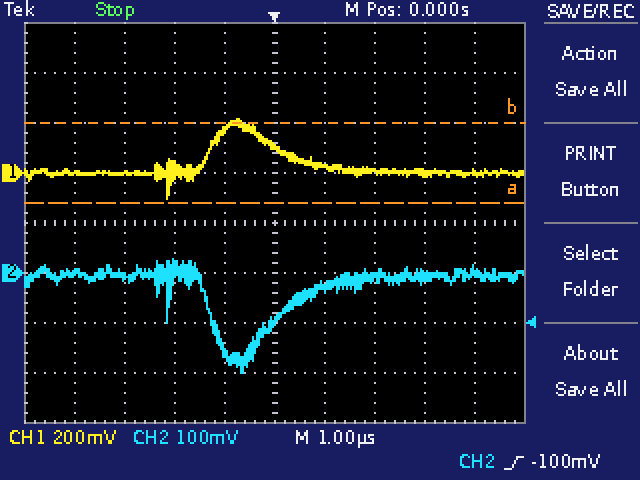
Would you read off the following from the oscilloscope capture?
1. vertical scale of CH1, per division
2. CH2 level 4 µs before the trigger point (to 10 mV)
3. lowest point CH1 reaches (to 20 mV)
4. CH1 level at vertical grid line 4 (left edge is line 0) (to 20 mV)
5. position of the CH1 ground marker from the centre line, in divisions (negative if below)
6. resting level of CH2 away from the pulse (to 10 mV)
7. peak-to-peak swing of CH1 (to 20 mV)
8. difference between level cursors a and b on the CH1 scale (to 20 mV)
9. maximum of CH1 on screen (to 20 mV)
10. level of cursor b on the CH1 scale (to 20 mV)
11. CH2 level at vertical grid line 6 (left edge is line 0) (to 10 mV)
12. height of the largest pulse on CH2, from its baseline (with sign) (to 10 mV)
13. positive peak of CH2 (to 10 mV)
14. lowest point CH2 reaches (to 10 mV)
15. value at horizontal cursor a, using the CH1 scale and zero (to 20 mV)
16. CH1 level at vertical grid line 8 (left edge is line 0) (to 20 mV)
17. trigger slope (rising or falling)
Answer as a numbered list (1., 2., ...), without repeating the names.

1. 200 mV
2. 0 mV
3. -100 mV
4. 180 mV
5. +1.0 div
6. -10 mV
7. 320 mV
8. 320 mV
9. 220 mV
10. 200 mV
11. -30 mV
12. -190 mV
13. 30 mV
14. -200 mV
15. -120 mV
16. 0 mV
17. rising
